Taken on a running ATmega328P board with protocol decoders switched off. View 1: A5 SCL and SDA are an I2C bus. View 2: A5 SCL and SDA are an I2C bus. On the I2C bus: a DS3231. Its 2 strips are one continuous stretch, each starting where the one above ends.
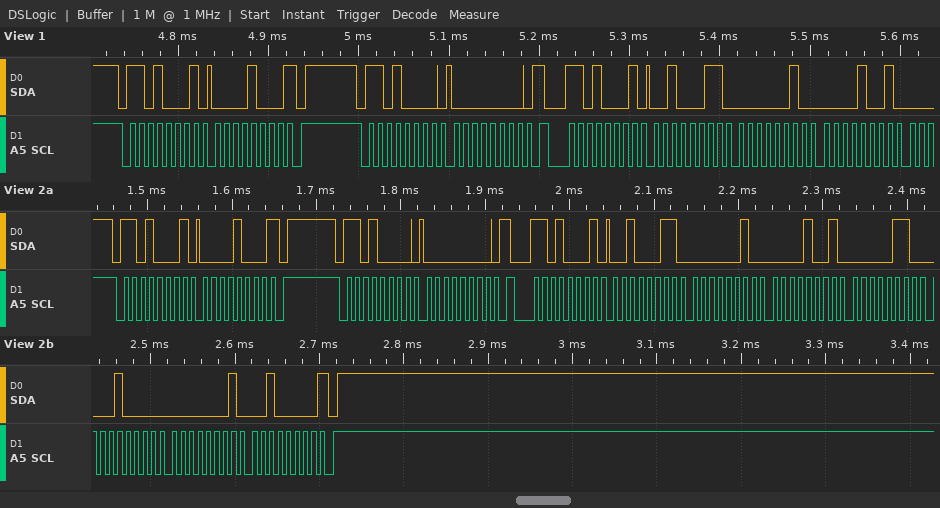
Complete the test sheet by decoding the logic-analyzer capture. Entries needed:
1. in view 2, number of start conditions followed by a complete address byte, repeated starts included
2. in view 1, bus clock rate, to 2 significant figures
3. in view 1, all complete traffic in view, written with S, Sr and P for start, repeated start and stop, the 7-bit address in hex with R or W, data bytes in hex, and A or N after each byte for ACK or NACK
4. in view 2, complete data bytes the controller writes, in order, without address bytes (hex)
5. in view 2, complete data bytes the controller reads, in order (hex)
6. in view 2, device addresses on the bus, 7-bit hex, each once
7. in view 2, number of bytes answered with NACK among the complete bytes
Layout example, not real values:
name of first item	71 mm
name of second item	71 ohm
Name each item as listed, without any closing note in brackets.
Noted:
in view 2, number of start conditions followed by a complete address byte, repeated starts included	3
in view 1, bus clock rate, to 2 significant figures	100 kHz
in view 1, all complete traffic in view, written with S, Sr and P for start, repeated start and stop, the 7-bit address in hex with R or W, data bytes in hex, and A or N after each byte for ACK or NACK	S 68R A 08 N P S 68W A 00 A Sr 68R A 23 A 02 A 09 A
in view 2, complete data bytes the controller writes, in order, without address bytes	00
in view 2, complete data bytes the controller reads, in order	08 23 02 09 06 10 01 20
in view 2, device addresses on the bus, 7-bit hex, each once	0x68
in view 2, number of bytes answered with NACK among the complete bytes	2
